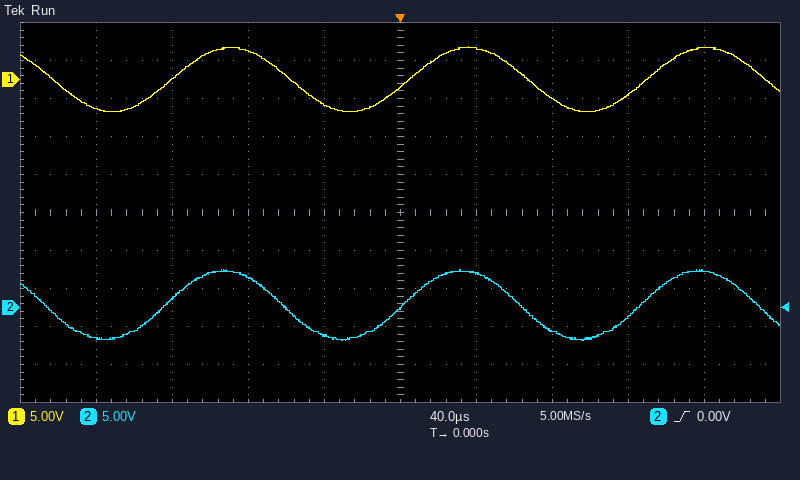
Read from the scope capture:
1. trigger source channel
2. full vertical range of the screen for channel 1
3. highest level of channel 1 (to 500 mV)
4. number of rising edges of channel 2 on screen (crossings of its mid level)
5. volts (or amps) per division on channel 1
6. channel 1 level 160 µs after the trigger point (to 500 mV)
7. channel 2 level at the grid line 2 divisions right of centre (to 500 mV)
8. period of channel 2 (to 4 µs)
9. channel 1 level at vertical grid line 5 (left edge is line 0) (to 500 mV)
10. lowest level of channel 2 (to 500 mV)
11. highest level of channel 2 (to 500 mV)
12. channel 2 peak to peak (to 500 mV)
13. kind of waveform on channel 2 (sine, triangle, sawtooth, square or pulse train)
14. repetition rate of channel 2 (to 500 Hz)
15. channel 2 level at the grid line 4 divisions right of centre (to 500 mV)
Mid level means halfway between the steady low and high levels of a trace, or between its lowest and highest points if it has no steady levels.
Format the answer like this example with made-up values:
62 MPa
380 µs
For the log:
channel 2
50 V
4.5 V
3
5 V
4.0 V
-3.0 V
124 µs
-1.0 V
-4.5 V
5.0 V
9.5 V
sine
8.0 kHz
5.0 V
